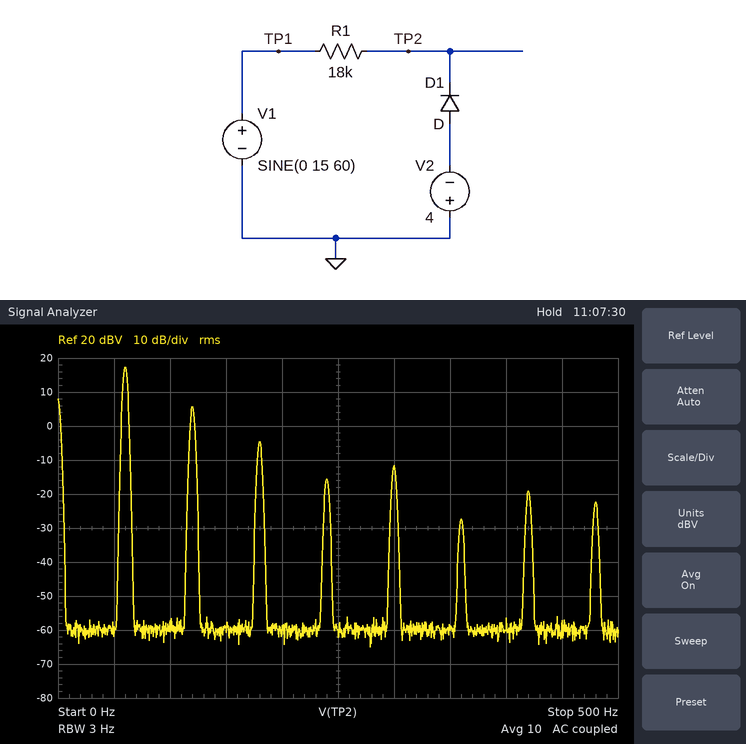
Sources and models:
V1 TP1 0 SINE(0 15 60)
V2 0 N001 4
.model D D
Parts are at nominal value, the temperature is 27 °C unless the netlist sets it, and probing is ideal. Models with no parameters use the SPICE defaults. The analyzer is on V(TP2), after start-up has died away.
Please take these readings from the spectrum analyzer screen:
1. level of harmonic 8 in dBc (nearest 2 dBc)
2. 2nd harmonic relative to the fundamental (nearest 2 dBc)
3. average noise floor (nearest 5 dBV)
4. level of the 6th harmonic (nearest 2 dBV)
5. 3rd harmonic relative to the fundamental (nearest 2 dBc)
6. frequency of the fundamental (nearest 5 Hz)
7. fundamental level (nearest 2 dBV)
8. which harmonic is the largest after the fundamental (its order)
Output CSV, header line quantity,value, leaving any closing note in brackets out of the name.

quantity,value
level of harmonic 8 in dBc,-40 dBc
2nd harmonic relative to the fundamental,-12 dBc
average noise floor,-60 dBV
level of the 6th harmonic,-28 dBV
3rd harmonic relative to the fundamental,-22 dBc
frequency of the fundamental,60 Hz
fundamental level,18 dBV
which harmonic is the largest after the fundamental,2
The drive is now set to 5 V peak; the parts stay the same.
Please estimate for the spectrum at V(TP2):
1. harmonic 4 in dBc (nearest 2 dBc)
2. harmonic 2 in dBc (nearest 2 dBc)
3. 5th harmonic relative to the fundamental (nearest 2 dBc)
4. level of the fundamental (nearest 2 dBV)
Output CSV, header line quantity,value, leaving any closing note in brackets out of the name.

quantity,value
harmonic 4 in dBc,-38 dBc
harmonic 2 in dBc,-36 dBc
5th harmonic relative to the fundamental,-40 dBc
level of the fundamental,10 dBV
